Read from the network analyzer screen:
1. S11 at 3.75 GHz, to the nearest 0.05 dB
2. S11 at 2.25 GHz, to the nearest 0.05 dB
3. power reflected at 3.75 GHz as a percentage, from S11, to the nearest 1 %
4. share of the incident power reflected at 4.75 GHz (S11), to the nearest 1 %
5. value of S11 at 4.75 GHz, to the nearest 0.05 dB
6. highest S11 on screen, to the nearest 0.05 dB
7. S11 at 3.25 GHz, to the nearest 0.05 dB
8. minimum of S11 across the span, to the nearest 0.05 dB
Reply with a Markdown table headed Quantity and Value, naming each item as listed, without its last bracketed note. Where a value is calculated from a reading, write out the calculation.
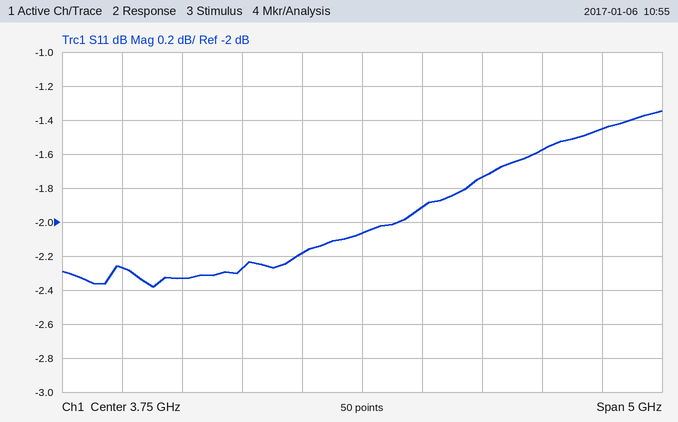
| Quantity | Value |
|---|---|
| S11 at 3.75 GHz, to the nearest 0.05 dB | -2.05 dB |
| S11 at 2.25 GHz, to the nearest 0.05 dB | -2.35 dB |
| power reflected at 3.75 GHz as a percentage, from S11, to the nearest 1 % | 10^(-2.05/10) ≈ 62 % |
| share of the incident power reflected at 4.75 GHz (S11), to the nearest 1 % | 10^(-1.75/10) ≈ 67 % |
| value of S11 at 4.75 GHz, to the nearest 0.05 dB | -1.75 dB |
| highest S11 on screen, to the nearest 0.05 dB | -1.35 dB |
| S11 at 3.25 GHz, to the nearest 0.05 dB | -2.20 dB |
| minimum of S11 across the span, to the nearest 0.05 dB | -2.40 dB |
